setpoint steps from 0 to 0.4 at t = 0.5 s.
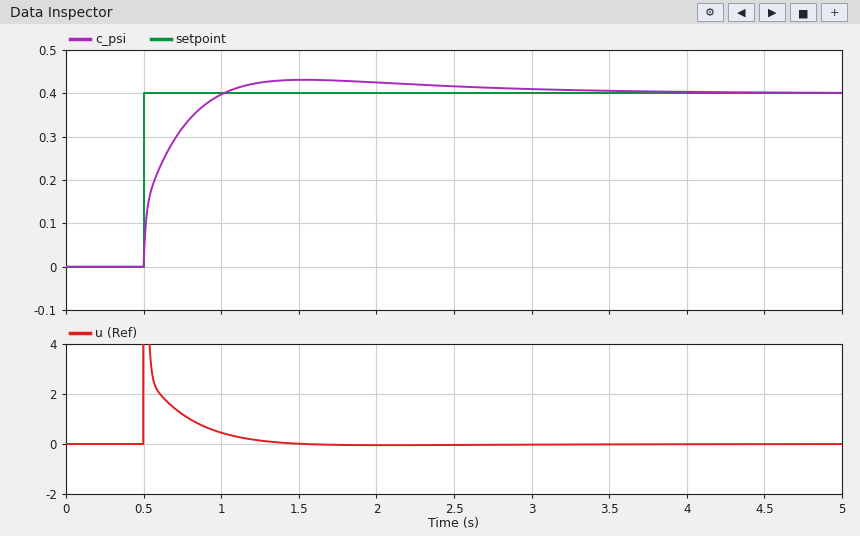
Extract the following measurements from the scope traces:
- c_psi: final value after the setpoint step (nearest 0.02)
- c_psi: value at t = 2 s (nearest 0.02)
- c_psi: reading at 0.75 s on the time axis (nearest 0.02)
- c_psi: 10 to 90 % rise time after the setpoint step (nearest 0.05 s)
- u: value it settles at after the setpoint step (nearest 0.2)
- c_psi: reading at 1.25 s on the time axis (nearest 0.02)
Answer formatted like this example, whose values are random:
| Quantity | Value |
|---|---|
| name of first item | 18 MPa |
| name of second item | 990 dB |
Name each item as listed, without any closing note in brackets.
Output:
| Quantity | Value |
|---|---|
| c_psi: final value after the setpoint step | 0.40 |
| c_psi: value at t = 2 s | 0.42 |
| c_psi: reading at 0.75 s on the time axis | 0.32 |
| c_psi: 10 to 90 % rise time after the setpoint step | 0.35 s |
| u: value it settles at after the setpoint step | 0.0 |
| c_psi: reading at 1.25 s on the time axis | 0.42 |
